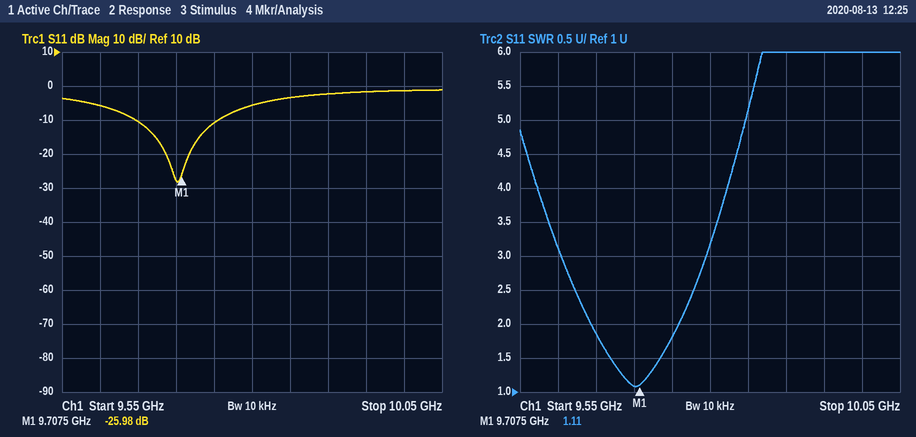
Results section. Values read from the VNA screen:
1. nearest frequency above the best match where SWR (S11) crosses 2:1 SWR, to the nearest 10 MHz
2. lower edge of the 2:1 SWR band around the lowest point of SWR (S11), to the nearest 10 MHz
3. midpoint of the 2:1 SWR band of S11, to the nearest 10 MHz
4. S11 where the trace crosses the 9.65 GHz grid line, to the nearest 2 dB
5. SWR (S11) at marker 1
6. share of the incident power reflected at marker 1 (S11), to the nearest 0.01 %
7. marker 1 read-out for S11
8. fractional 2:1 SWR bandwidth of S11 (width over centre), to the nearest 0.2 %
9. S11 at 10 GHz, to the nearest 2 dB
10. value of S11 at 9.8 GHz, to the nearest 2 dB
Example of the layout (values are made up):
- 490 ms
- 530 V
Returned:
- 9.76 GHz
- 9.64 GHz
- 9.70 GHz
- -10 dB
- 1.11
- 0.25 %
- -25.98 dB
- 1.2 %
- -2 dB
- -6 dB
